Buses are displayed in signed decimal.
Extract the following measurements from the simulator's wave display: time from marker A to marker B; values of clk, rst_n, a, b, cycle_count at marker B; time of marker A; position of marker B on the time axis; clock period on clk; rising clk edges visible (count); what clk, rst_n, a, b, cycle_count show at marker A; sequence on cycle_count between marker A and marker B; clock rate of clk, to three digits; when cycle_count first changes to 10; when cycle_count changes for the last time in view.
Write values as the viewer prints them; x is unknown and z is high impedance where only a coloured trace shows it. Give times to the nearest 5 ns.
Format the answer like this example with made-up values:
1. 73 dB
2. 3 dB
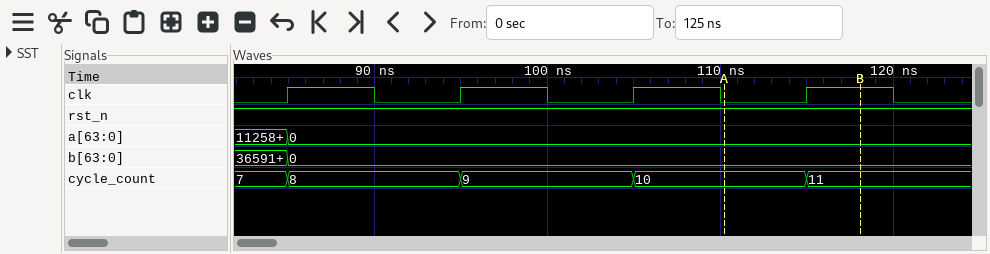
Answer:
1. 10 ns
2. clk=1, rst_n=1, a=0, b=0, cycle_count=11
3. 110 ns
4. 120 ns
5. 10 ns
6. 4
7. clk=0, rst_n=1, a=0, b=0, cycle_count=10
8. 10, 11
9. 100 MHz
10. 105 ns
11. 115 ns
